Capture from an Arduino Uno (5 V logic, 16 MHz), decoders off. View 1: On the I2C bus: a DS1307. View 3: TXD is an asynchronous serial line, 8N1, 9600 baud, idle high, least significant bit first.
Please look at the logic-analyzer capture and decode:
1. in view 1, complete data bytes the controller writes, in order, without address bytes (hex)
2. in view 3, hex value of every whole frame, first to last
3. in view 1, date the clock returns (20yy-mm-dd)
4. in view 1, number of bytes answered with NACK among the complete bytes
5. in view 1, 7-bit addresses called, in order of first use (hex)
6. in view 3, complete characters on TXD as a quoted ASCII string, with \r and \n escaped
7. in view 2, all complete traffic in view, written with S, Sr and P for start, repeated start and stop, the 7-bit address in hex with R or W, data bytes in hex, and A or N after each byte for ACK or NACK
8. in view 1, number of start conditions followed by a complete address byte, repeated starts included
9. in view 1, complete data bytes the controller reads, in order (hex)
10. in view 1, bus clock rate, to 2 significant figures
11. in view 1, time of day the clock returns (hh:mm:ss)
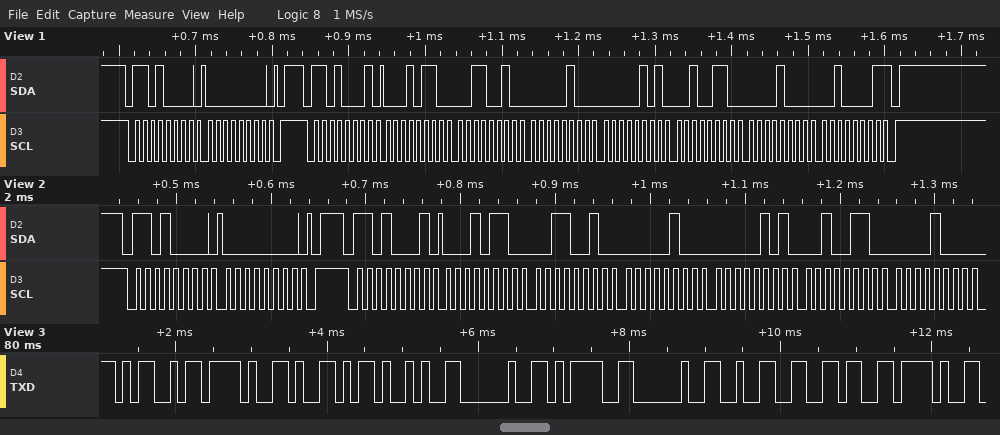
00
4D 2F 59 29 20 3D 20 32 36 2F
2021-08-26
1
0x68
"M/Y) = 26/"
S 68W A 00 A P S 68R A 16 A 32 A 04 A 05 A 26 A 08 A
2
16 32 04 05 26 08 21
100 kHz
04:32:16
